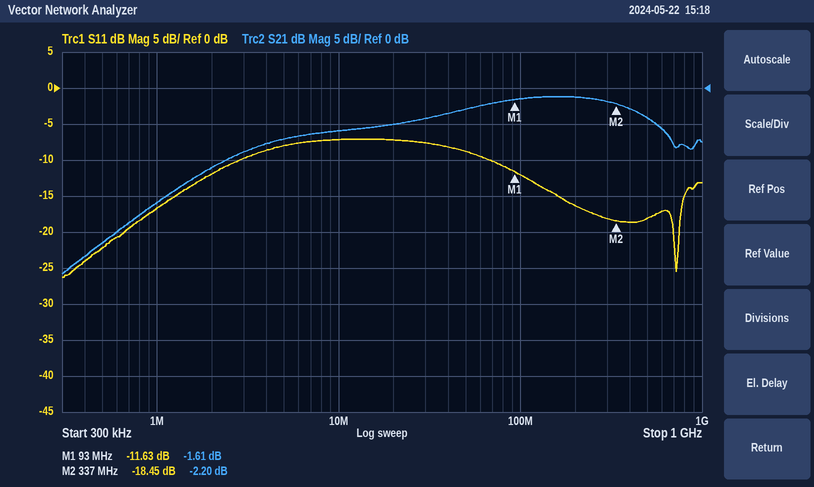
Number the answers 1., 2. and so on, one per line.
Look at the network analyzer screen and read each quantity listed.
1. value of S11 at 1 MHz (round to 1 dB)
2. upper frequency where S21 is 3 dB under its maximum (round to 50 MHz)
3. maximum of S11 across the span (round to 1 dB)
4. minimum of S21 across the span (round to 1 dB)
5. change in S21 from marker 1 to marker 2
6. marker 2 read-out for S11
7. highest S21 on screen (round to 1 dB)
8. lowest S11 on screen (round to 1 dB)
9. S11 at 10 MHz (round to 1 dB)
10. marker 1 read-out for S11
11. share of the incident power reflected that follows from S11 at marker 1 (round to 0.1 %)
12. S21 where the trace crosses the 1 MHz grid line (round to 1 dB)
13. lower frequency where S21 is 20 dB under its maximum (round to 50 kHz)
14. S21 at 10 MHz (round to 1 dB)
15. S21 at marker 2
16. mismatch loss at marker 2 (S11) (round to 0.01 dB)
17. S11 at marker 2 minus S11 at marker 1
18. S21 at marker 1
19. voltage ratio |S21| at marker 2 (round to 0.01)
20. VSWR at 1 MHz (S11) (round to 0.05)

1. -17 dB
2. 500 MHz
3. -7 dB
4. -26 dB
5. -0.59 dB
6. -18.45 dB
7. -1 dB
8. -26 dB
9. -7 dB
10. -11.63 dB
11. 6.9 %
12. -16 dB
13. 500 kHz
14. -6 dB
15. -2.20 dB
16. 0.06 dB
17. -6.82 dB
18. -1.61 dB
19. 0.78
20. 1.35
